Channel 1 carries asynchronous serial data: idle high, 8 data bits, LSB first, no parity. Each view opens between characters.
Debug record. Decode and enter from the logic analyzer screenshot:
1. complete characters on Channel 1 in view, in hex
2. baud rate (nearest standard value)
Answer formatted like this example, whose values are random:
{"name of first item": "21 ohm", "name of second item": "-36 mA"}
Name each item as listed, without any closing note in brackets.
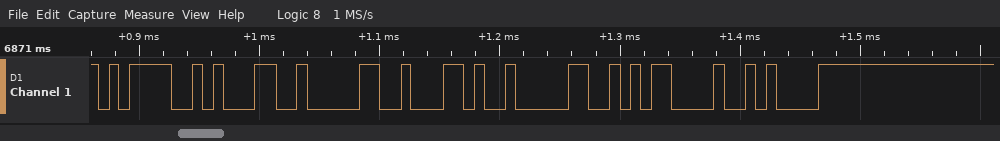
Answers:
{"complete characters on Channel 1 in view, in hex": "3D, 31, 30, 2C, 30, 0D, 0A", "baud rate": "115200 baud"}
